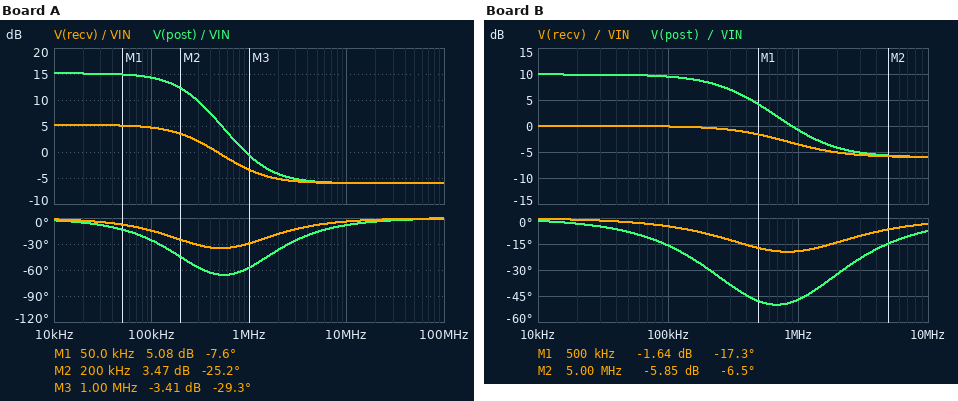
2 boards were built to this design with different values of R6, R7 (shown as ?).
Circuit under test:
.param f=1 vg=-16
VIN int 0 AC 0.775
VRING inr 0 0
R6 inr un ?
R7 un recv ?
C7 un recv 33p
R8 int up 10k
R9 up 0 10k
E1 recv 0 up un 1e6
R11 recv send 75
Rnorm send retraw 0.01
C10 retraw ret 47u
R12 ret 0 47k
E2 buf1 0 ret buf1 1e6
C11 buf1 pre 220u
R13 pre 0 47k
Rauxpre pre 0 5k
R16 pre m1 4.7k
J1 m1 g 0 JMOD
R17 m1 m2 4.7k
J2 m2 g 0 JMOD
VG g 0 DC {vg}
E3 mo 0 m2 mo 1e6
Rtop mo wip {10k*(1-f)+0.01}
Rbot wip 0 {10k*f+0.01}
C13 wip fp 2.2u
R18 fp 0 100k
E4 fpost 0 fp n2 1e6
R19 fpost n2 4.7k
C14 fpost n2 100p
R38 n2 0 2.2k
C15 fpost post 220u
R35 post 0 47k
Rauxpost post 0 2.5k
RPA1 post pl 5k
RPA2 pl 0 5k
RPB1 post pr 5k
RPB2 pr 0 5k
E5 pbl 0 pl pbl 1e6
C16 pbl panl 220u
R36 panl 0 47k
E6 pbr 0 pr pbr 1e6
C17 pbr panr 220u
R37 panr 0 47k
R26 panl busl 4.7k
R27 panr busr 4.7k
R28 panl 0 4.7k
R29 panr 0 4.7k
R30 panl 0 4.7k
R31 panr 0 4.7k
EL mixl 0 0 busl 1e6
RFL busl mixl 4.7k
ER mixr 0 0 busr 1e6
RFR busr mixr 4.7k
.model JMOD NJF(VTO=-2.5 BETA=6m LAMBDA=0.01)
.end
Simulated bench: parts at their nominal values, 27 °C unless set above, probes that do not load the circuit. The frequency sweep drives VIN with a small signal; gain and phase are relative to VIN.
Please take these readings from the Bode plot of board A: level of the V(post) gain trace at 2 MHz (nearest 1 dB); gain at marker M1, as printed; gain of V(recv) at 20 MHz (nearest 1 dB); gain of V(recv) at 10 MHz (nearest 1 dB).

-4 dB
5.08 dB
-6 dB
-6 dB
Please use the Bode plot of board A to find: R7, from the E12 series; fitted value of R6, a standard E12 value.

18 kΩ
6.8 kΩ
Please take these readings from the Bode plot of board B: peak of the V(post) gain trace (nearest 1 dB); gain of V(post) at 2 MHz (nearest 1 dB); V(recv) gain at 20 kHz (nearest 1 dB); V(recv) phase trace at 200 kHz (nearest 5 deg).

10 dB
-4 dB
0 dB
-10 deg
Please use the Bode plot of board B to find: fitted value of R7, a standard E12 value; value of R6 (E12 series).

8.2 kΩ
8.2 kΩ
